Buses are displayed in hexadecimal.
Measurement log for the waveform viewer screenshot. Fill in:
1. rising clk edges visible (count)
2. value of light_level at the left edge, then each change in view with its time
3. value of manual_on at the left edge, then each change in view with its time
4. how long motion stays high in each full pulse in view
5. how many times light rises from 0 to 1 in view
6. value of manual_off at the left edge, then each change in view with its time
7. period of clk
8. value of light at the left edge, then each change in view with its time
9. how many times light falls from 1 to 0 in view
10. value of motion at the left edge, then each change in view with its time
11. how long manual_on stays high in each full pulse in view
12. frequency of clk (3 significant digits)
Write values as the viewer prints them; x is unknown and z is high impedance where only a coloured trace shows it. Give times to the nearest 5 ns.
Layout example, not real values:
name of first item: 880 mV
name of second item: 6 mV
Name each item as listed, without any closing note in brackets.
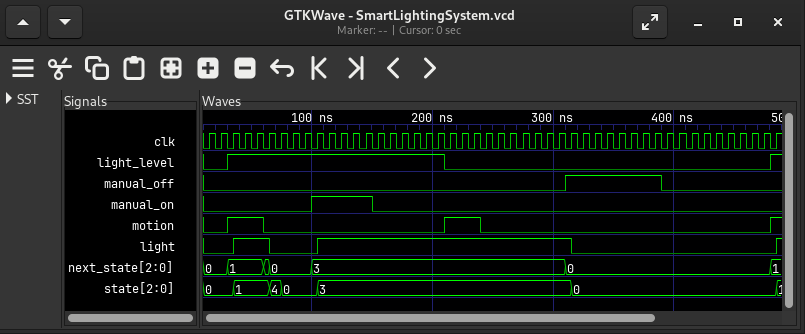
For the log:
rising clk edges visible: 48
value of light_level at the left edge, then each change in view with its time: 0, 1 at 30 ns, 0 at 210 ns, 1 at 480 ns
value of manual_on at the left edge, then each change in view with its time: 0, 1 at 100 ns, 0 at 150 ns
how long motion stays high in each full pulse in view: 30 ns, 30 ns
how many times light rises from 0 to 1 in view: 3
value of manual_off at the left edge, then each change in view with its time: 0, 1 at 310 ns, 0 at 390 ns
period of clk: 10 ns
value of light at the left edge, then each change in view with its time: 0, 1 at 35 ns, 0 at 65 ns, 1 at 105 ns, 0 at 315 ns, 1 at 485 ns
how many times light falls from 1 to 0 in view: 2
value of motion at the left edge, then each change in view with its time: 0, 1 at 30 ns, 0 at 60 ns, 1 at 210 ns, 0 at 240 ns, 1 at 480 ns
how long manual_on stays high in each full pulse in view: 50 ns
frequency of clk: 100 MHz
